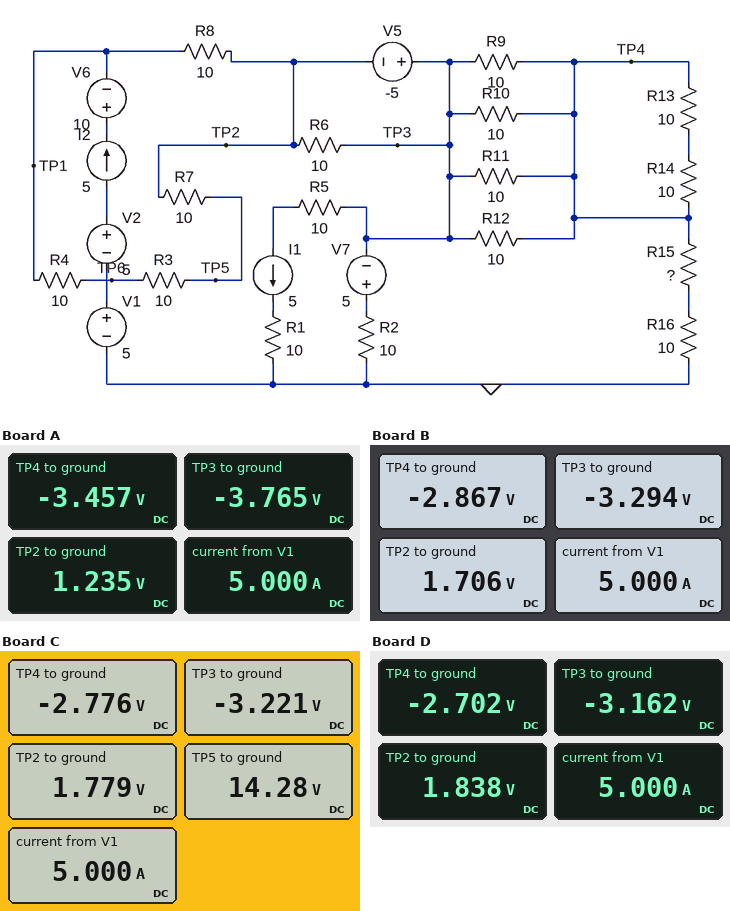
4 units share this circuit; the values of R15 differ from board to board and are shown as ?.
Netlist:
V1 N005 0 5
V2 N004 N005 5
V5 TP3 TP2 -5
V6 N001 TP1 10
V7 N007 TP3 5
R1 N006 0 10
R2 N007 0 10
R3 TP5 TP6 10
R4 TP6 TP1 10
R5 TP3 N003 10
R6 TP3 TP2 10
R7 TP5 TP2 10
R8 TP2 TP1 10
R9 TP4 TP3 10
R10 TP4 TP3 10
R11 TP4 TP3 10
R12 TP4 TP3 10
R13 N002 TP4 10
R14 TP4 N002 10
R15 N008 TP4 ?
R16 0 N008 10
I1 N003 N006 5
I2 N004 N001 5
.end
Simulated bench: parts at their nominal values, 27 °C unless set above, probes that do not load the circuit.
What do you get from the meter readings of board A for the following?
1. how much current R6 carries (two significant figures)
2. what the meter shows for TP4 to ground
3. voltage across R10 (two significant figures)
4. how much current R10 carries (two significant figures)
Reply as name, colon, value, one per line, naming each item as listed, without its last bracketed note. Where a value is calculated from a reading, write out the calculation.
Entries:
how much current R6 carries: (1.235 V - (-3.765 V)) / 10 Ω = 500 mA
what the meter shows for TP4 to ground: -3.457 V
voltage across R10: -3.457 V - (-3.765 V) = 310 mV
how much current R10 carries: (-3.457 V - (-3.765 V)) / 10 Ω = 31 mA
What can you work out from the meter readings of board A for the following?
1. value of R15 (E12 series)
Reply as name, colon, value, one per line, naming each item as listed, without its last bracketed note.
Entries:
value of R15: 18 Ω
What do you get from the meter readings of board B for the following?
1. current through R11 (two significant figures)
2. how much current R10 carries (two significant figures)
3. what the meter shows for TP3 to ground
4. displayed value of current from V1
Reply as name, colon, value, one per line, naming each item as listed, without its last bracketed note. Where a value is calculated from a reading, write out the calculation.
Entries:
current through R11: (-2.867 V - (-3.294 V)) / 10 Ω = 43 mA
how much current R10 carries: (-2.867 V - (-3.294 V)) / 10 Ω = 43 mA
what the meter shows for TP3 to ground: -3.294 V
displayed value of current from V1: 5.000 A
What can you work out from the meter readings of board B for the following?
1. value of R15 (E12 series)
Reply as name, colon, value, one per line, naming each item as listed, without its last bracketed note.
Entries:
value of R15: 6.8 Ω
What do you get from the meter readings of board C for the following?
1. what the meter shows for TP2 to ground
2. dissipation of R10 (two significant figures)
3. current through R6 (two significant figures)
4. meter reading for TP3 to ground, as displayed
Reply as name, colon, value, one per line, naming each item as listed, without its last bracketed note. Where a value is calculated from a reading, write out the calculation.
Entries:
what the meter shows for TP2 to ground: 1.779 V
dissipation of R10: (-2.776 V - (-3.221 V))^2 / 10 Ω = 20 mW
current through R6: (1.779 V - (-3.221 V)) / 10 Ω = 500 mA
meter reading for TP3 to ground, as displayed: -3.221 V
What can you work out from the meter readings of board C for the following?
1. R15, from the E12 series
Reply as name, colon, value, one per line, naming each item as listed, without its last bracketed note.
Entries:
R15, from the E12 series: 5.6 Ω
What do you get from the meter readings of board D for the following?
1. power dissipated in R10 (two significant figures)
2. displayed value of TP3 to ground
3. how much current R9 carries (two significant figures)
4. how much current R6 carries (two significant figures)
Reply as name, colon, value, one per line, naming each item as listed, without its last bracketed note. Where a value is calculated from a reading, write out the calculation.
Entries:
power dissipated in R10: (-2.702 V - (-3.162 V))^2 / 10 Ω = 21 mW
displayed value of TP3 to ground: -3.162 V
how much current R9 carries: (-2.702 V - (-3.162 V)) / 10 Ω = 46 mA
how much current R6 carries: (1.838 V - (-3.162 V)) / 10 Ω = 500 mA
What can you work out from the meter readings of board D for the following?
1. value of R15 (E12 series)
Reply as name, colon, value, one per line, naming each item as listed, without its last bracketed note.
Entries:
value of R15: 4.7 Ω
